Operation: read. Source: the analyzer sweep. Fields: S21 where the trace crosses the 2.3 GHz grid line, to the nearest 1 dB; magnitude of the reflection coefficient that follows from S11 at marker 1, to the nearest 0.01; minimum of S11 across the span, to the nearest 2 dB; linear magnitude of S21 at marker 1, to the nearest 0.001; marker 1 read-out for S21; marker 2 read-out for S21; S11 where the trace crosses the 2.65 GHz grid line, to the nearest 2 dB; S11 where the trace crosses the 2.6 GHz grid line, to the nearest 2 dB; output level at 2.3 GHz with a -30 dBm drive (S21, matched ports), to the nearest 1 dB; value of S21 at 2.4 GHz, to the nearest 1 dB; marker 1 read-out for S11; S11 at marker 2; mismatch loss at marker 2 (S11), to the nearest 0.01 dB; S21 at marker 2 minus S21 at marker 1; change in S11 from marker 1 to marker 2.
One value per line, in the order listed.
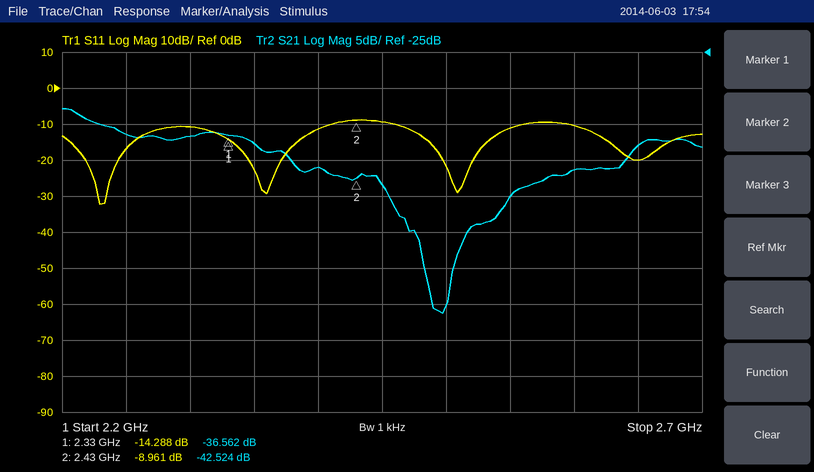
-37 dB
0.19
-32 dB
0.015
-36.562 dB
-42.524 dB
-20 dB
-10 dB
-67 dBm
-41 dB
-14.288 dB
-8.961 dB
0.59 dB
-5.962 dB
5.327 dB
